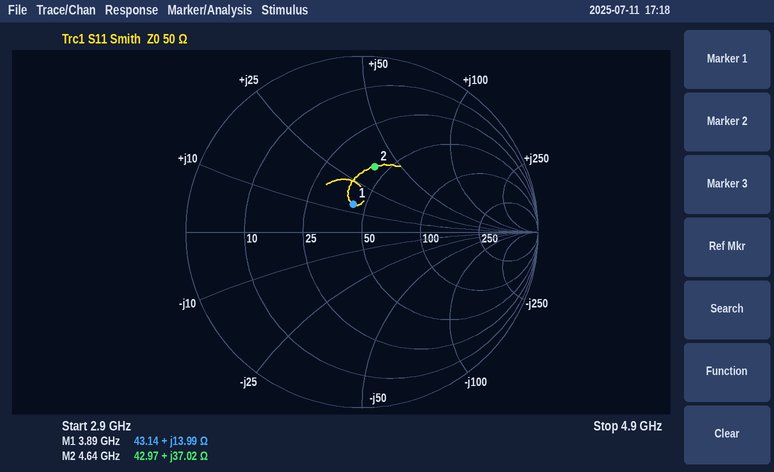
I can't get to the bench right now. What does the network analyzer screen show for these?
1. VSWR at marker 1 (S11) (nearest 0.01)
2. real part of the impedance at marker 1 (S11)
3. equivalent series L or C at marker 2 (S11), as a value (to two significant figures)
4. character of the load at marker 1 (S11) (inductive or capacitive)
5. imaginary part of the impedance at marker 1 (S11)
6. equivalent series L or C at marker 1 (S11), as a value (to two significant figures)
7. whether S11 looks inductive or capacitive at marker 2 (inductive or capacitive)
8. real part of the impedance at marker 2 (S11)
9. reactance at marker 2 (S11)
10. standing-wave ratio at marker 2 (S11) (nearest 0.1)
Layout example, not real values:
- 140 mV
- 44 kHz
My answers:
- 1.40
- 43.14 Ω
- 1.3 nH
- inductive
- +13.99 Ω
- 570 pH
- inductive
- 42.97 Ω
- +37.02 Ω
- 2.2
